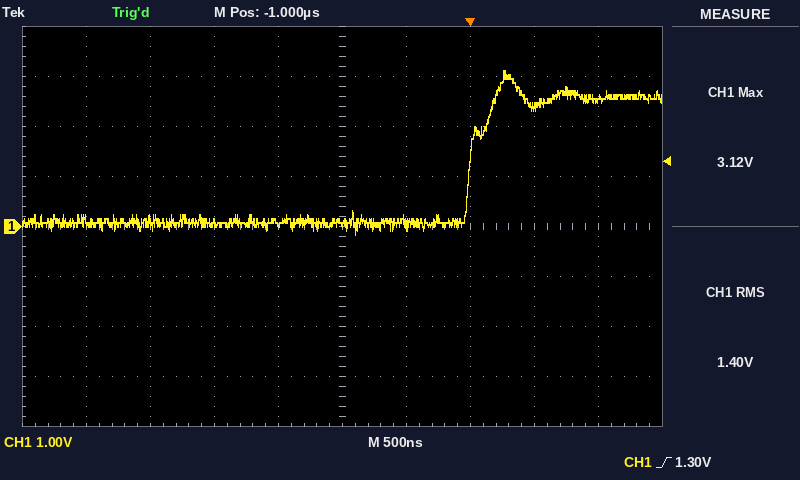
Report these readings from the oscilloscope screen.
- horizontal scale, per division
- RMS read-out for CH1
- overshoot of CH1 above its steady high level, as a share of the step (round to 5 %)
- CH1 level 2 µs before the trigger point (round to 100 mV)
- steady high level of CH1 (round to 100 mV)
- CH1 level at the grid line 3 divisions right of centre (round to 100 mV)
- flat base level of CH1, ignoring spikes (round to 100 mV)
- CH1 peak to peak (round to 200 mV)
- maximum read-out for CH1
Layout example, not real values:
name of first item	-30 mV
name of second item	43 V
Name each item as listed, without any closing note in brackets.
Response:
horizontal scale, per division	500 ns
RMS read-out for CH1	1.40 V
overshoot of CH1 above its steady high level, as a share of the step	20 %
CH1 level 2 µs before the trigger point	100 mV
steady high level of CH1	2.6 V
CH1 level at the grid line 3 divisions right of centre	2.4 V
flat base level of CH1, ignoring spikes	100 mV
CH1 peak to peak	3.2 V
maximum read-out for CH1	3.12 V
